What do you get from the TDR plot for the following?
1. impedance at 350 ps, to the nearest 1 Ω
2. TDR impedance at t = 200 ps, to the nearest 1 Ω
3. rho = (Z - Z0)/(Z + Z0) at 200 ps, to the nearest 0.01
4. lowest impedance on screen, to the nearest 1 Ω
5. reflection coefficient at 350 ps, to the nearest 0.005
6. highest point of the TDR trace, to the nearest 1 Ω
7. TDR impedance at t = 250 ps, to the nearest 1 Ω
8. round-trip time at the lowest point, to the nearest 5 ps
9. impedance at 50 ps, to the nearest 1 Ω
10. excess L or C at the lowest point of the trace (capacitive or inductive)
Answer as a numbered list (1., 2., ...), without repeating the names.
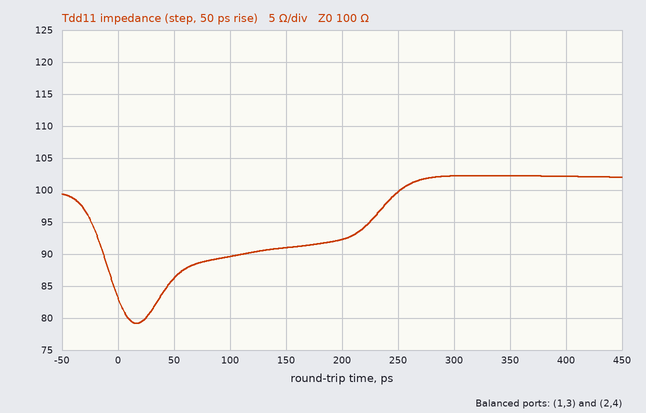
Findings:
1. 102 Ω
2. 92 Ω
3. -0.04
4. 79 Ω
5. +0.010
6. 102 Ω
7. 100 Ω
8. 15 ps
9. 86 Ω
10. capacitive
